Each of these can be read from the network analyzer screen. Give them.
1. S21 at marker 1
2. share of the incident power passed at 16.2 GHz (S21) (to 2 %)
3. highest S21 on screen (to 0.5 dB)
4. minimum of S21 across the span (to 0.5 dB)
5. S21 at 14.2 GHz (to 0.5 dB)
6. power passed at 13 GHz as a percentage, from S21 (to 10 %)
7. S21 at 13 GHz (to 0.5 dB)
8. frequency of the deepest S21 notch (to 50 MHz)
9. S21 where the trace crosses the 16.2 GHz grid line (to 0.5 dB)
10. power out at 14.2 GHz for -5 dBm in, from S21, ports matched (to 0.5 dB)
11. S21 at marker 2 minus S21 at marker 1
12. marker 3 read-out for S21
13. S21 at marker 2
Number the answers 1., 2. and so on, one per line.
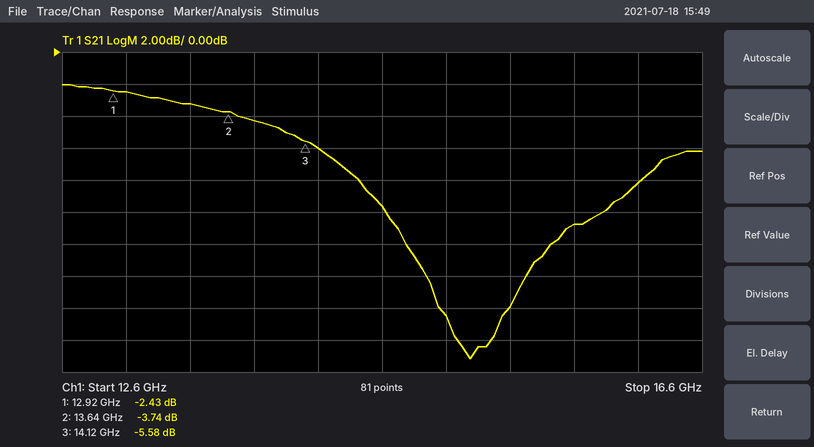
1. -2.43 dB
2. 16 %
3. -2.0 dB
4. -19.0 dB
5. -6.0 dB
6. 60 %
7. -2.5 dB
8. 15.15 GHz
9. -8.0 dB
10. -11.0 dBm
11. -1.31 dB
12. -5.58 dB
13. -3.74 dB
